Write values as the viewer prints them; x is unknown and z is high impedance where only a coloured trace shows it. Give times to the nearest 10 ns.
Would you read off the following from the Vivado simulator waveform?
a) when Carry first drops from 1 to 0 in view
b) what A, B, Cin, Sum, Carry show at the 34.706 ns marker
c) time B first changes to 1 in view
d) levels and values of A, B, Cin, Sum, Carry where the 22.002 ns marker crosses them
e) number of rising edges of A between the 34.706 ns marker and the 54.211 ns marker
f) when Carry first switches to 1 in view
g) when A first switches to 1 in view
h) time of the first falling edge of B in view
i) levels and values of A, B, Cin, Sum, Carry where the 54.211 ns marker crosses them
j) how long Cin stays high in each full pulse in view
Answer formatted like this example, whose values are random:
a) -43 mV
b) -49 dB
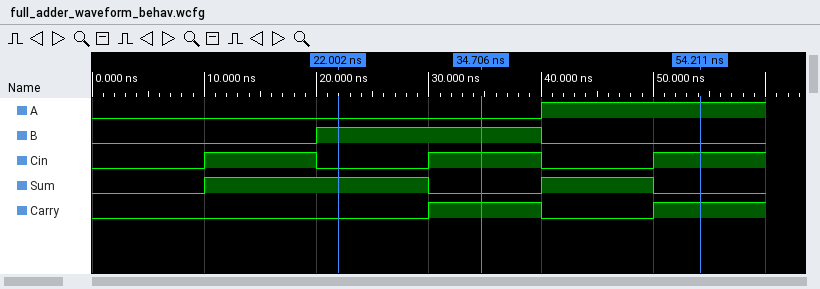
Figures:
a) 40 ns
b) A=0, B=1, Cin=1, Sum=0, Carry=1
c) 20 ns
d) A=0, B=1, Cin=0, Sum=1, Carry=0
e) 1
f) 30 ns
g) 40 ns
h) 40 ns
i) A=1, B=0, Cin=1, Sum=0, Carry=1
j) 10 ns, 10 ns
